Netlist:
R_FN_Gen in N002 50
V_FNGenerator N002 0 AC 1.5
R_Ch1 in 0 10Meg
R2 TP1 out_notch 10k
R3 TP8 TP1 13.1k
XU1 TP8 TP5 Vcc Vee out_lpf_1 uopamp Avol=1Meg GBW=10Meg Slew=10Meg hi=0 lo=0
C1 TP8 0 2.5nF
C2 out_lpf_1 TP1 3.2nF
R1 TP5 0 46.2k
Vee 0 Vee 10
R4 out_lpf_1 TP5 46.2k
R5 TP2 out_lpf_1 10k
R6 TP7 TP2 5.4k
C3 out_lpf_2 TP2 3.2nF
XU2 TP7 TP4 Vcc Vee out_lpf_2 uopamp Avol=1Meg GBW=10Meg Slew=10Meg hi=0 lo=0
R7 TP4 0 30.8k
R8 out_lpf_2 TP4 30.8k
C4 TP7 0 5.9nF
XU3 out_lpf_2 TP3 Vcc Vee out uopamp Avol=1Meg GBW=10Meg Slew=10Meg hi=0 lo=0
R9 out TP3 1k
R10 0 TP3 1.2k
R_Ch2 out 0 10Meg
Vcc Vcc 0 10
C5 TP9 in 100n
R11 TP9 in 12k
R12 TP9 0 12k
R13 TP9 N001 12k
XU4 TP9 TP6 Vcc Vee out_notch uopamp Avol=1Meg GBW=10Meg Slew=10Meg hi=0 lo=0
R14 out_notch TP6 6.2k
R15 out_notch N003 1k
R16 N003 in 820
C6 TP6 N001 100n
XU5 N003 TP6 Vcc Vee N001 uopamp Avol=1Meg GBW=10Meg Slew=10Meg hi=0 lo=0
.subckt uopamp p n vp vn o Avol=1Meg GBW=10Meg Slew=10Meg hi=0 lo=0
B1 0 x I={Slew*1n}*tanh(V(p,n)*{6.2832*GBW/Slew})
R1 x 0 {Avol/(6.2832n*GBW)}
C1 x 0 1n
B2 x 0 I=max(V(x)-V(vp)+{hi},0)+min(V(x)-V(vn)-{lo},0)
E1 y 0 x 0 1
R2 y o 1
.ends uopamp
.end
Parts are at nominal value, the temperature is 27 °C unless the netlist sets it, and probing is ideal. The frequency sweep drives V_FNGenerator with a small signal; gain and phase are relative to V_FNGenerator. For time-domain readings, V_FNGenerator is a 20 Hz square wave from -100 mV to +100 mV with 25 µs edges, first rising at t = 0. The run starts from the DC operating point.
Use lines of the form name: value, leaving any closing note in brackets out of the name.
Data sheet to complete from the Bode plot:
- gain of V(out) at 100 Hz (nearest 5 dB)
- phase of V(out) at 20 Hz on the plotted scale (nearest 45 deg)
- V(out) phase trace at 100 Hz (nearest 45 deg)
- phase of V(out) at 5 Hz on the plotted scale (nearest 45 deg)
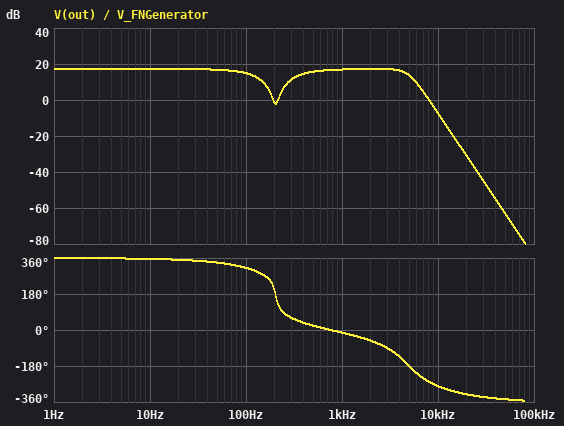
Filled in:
gain of V(out) at 100 Hz: 15 dB
phase of V(out) at 20 Hz on the plotted scale: 360 deg
V(out) phase trace at 100 Hz: 315 deg
phase of V(out) at 5 Hz on the plotted scale: 360 deg
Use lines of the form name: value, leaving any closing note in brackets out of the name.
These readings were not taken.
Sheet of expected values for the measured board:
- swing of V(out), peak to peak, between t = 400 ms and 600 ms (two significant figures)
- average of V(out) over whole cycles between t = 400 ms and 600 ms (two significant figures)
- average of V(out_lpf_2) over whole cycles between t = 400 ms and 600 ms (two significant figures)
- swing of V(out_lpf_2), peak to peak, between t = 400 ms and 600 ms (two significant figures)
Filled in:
swing of V(out), peak to peak, between t = 400 ms and 600 ms: 1.6 V
average of V(out) over whole cycles between t = 400 ms and 600 ms: 94 mV
average of V(out_lpf_2) over whole cycles between t = 400 ms and 600 ms: 51 mV
swing of V(out_lpf_2), peak to peak, between t = 400 ms and 600 ms: 870 mV
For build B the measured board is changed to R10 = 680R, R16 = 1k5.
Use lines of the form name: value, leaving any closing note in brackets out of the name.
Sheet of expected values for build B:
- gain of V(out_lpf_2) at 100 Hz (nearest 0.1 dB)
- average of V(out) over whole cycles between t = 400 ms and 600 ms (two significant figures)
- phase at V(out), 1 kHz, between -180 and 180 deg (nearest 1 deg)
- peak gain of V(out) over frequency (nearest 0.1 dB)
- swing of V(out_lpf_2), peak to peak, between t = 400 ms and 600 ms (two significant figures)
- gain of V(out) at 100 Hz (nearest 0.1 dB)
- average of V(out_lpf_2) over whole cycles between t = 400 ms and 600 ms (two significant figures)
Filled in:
gain of V(out_lpf_2) at 100 Hz: 5.1 dB
average of V(out) over whole cycles between t = 400 ms and 600 ms: 120 mV
phase at V(out), 1 kHz, between -180 and 180 deg: -18 deg
peak gain of V(out) over frequency: 19.9 dB
swing of V(out_lpf_2), peak to peak, between t = 400 ms and 600 ms: 800 mV
gain of V(out) at 100 Hz: 13.0 dB
average of V(out_lpf_2) over whole cycles between t = 400 ms and 600 ms: 49 mV
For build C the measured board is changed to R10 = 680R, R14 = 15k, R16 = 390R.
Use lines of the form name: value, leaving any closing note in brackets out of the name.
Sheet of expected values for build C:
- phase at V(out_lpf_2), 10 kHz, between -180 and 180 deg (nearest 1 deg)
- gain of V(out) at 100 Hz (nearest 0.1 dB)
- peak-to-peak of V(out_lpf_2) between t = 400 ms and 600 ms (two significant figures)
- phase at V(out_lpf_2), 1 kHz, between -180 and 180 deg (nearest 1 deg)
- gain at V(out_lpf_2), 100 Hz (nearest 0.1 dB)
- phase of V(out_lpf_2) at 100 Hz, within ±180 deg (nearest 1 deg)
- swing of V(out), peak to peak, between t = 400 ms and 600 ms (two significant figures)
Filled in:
phase at V(out_lpf_2), 10 kHz, between -180 and 180 deg: 80 deg
gain of V(out) at 100 Hz: 18.7 dB
peak-to-peak of V(out_lpf_2) between t = 400 ms and 600 ms: 1.0 V
phase at V(out_lpf_2), 1 kHz, between -180 and 180 deg: -2 deg
gain at V(out_lpf_2), 100 Hz: 10.8 dB
phase of V(out_lpf_2) at 100 Hz, within ±180 deg: -89 deg
swing of V(out), peak to peak, between t = 400 ms and 600 ms: 2.5 V
